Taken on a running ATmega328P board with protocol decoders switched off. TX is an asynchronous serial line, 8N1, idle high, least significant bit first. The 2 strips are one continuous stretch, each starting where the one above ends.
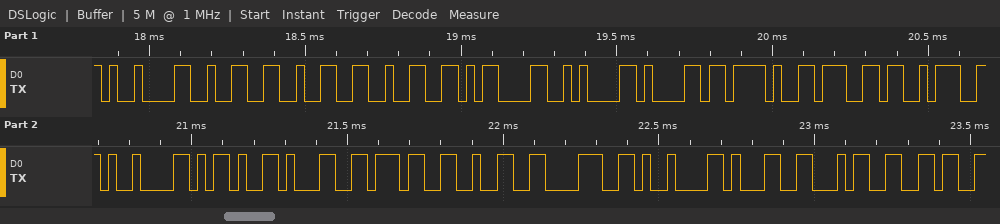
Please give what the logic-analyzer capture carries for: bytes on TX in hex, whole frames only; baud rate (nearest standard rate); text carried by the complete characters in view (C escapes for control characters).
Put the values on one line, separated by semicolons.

09 32 32 32 0D 0A 61 2F 67 3A 09 2D 31 37 32 38 09 31 34 36; 38400 baud; "\t222\r\na/g:\t-1728\t146"
